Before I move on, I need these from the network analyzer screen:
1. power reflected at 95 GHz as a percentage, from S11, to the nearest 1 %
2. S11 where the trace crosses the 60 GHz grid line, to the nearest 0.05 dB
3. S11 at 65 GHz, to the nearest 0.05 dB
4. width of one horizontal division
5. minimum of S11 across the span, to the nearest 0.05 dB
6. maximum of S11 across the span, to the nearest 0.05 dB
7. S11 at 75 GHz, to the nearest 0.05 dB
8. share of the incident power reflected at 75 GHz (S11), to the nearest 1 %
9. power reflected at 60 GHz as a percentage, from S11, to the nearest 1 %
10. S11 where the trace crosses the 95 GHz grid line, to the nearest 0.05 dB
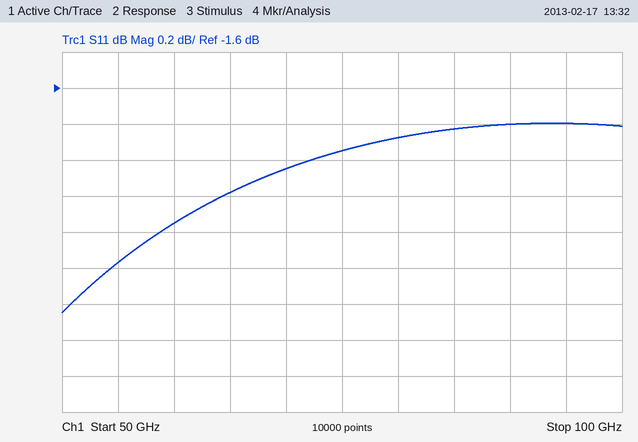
66 %
-2.35 dB
-2.20 dB
5 GHz
-2.85 dB
-1.80 dB
-1.95 dB
64 %
58 %
-1.80 dB
